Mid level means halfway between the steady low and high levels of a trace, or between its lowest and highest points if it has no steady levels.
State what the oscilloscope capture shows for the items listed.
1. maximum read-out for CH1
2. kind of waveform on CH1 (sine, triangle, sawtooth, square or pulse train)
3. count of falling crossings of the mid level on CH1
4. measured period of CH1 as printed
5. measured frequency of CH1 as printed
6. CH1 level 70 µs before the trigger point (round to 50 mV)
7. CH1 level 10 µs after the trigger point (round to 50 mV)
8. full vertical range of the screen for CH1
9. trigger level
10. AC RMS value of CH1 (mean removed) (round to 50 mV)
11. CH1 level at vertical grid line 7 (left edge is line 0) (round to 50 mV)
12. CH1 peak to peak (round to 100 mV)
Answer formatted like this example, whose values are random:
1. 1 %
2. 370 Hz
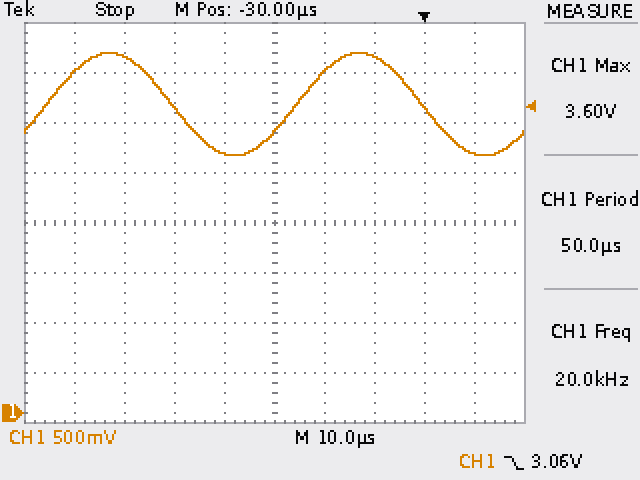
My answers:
1. 3.60 V
2. sine
3. 2
4. 50.0 µs
5. 20.0 kHz
6. 3.40 V
7. 2.60 V
8. 4 V
9. 3.06 V
10. 350 mV
11. 3.55 V
12. 1.00 V
